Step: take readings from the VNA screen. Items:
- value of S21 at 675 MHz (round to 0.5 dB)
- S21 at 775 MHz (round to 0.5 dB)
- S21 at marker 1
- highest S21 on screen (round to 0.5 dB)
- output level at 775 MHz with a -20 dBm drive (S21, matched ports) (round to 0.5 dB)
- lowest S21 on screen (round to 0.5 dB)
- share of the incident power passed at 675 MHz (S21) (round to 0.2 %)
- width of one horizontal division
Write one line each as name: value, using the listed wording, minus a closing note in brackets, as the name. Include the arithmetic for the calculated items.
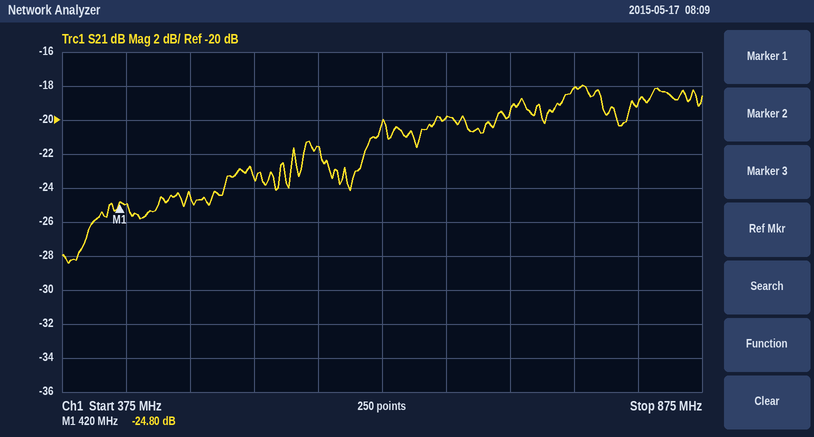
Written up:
value of S21 at 675 MHz: -20.0 dB
S21 at 775 MHz: -18.0 dB
S21 at marker 1: -24.80 dB
highest S21 on screen: -18.0 dB
output level at 775 MHz with a -20 dBm drive (S21, matched ports): -20 dBm + (-18.0 dB) = -38.0 dBm
lowest S21 on screen: -28.5 dB
share of the incident power passed at 675 MHz (S21): 10^(-20/10) ≈ 1.0 %
width of one horizontal division: 50 MHz
